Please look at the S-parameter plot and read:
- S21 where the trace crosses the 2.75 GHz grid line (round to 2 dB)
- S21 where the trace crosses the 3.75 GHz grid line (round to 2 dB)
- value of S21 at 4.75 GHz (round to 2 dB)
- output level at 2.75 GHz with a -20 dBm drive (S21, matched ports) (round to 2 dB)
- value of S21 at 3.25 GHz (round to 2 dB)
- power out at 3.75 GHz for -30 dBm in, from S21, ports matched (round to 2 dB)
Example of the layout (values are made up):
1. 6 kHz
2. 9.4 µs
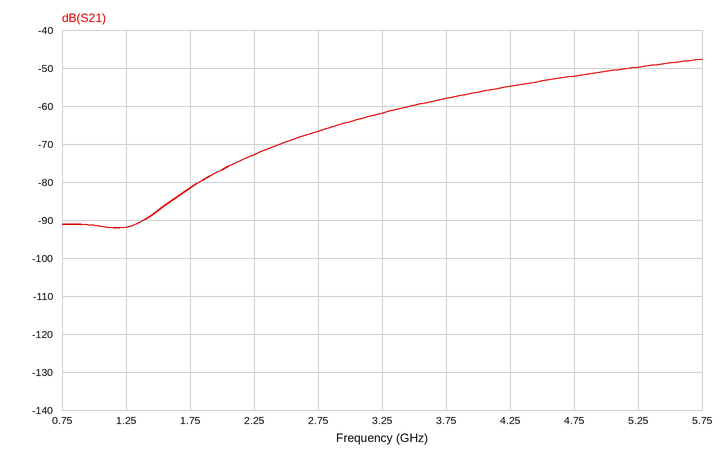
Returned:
1. -66 dB
2. -58 dB
3. -52 dB
4. -86 dBm
5. -62 dB
6. -88 dBm
